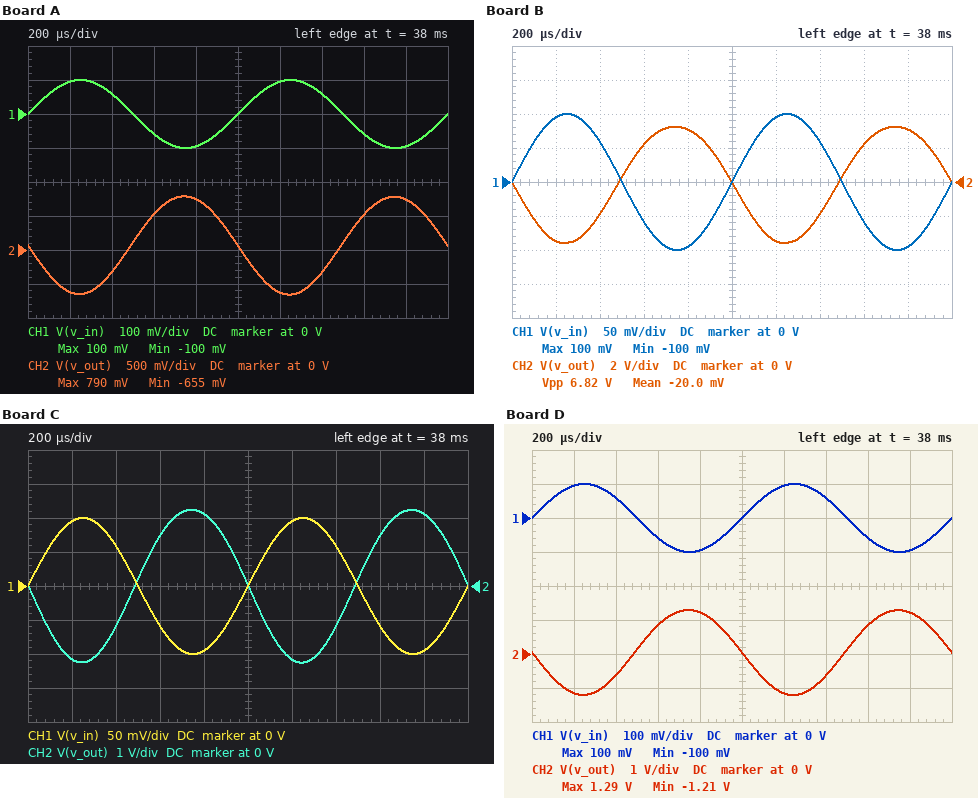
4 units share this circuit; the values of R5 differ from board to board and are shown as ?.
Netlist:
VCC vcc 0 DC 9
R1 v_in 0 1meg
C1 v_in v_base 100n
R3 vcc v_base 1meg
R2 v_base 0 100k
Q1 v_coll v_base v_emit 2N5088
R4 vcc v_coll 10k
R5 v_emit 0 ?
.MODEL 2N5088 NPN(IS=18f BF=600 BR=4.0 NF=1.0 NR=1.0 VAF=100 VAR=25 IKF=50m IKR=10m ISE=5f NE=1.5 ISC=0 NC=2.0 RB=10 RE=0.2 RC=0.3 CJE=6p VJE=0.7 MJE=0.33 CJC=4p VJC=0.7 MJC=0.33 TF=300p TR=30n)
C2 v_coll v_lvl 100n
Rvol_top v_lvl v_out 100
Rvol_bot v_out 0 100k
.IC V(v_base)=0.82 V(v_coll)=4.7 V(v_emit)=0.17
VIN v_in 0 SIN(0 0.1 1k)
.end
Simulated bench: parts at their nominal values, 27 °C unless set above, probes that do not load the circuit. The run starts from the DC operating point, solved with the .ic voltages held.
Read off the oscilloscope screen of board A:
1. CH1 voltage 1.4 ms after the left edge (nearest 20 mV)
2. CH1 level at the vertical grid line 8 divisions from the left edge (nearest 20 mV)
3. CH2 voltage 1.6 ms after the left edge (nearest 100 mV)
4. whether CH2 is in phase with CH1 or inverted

60 mV
-60 mV
500 mV
inverted
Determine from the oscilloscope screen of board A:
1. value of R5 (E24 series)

1.1 kΩ
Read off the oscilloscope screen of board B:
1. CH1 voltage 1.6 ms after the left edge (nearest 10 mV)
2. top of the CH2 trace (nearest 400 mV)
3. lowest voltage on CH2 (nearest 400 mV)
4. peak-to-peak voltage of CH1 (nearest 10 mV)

-60 mV
3.2 V
-3.6 V
200 mV
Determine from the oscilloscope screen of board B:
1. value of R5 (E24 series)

200 Ω
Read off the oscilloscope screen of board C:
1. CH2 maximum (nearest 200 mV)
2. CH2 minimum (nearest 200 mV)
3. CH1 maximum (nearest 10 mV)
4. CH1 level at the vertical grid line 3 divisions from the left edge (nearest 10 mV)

2.2 V
-2.2 V
100 mV
-60 mV
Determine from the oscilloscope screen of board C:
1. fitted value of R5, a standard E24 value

330 Ω
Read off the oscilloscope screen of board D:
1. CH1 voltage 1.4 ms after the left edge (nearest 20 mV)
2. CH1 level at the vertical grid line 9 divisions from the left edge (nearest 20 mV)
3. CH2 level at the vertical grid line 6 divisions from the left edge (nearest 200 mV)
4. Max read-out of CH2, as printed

60 mV
-100 mV
-1.2 V
1.29 V
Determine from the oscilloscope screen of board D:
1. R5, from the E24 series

620 Ω
